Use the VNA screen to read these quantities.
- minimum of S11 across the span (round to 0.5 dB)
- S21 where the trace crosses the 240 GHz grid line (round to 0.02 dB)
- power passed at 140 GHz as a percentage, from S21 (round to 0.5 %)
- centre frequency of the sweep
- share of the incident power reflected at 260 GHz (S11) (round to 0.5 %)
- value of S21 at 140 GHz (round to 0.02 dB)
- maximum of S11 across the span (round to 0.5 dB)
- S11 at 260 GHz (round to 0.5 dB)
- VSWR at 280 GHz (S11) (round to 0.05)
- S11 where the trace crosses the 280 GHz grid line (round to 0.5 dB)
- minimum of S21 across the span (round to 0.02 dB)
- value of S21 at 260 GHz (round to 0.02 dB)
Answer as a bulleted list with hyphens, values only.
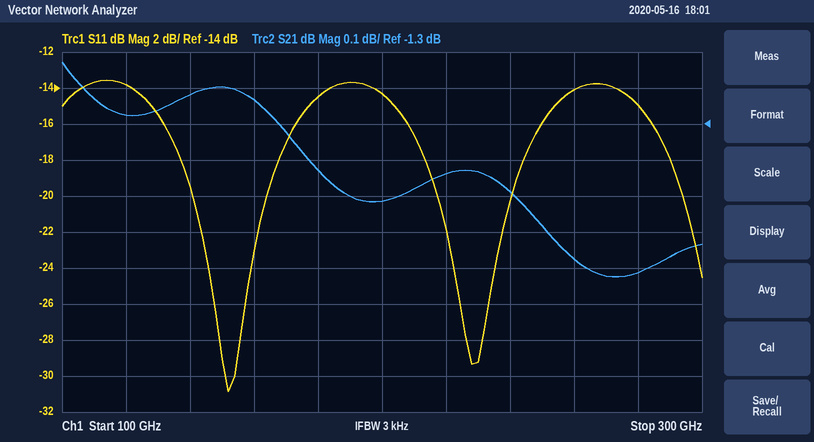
- -31.0 dB
- -1.48 dB
- 75.5 %
- 200 GHz
- 4.0 %
- -1.22 dB
- -13.5 dB
- -14.0 dB
- 1.45
- -15.0 dB
- -1.72 dB
- -1.68 dB
